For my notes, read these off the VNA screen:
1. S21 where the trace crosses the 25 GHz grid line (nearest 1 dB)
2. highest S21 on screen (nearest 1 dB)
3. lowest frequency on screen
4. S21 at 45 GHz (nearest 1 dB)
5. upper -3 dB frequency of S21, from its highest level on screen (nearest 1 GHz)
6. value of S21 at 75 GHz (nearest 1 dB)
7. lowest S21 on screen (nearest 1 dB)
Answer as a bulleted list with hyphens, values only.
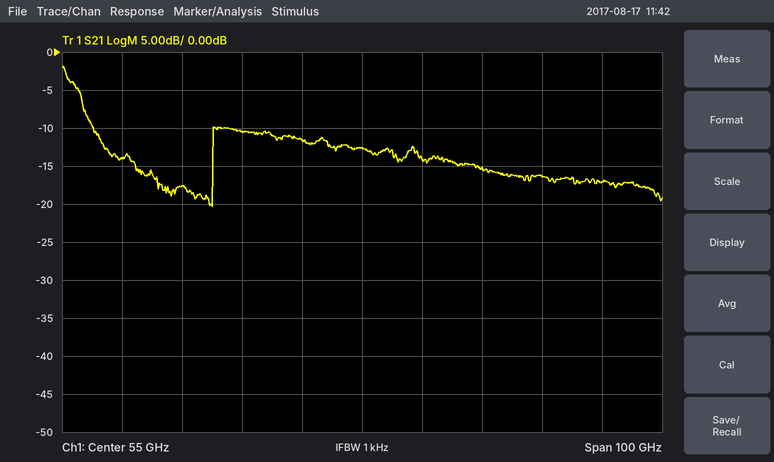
- -18 dB
- -2 dB
- 5 GHz
- -12 dB
- 8 GHz
- -15 dB
- -20 dB
